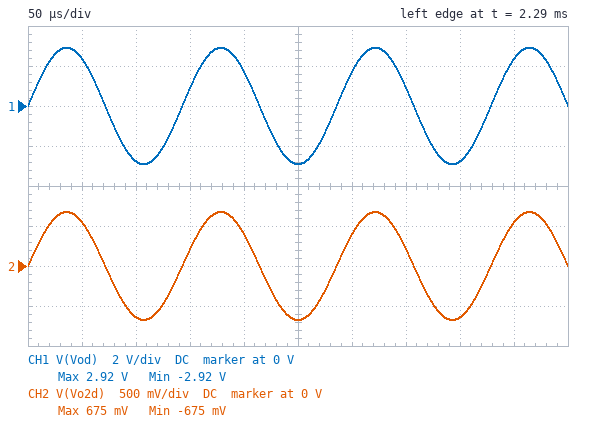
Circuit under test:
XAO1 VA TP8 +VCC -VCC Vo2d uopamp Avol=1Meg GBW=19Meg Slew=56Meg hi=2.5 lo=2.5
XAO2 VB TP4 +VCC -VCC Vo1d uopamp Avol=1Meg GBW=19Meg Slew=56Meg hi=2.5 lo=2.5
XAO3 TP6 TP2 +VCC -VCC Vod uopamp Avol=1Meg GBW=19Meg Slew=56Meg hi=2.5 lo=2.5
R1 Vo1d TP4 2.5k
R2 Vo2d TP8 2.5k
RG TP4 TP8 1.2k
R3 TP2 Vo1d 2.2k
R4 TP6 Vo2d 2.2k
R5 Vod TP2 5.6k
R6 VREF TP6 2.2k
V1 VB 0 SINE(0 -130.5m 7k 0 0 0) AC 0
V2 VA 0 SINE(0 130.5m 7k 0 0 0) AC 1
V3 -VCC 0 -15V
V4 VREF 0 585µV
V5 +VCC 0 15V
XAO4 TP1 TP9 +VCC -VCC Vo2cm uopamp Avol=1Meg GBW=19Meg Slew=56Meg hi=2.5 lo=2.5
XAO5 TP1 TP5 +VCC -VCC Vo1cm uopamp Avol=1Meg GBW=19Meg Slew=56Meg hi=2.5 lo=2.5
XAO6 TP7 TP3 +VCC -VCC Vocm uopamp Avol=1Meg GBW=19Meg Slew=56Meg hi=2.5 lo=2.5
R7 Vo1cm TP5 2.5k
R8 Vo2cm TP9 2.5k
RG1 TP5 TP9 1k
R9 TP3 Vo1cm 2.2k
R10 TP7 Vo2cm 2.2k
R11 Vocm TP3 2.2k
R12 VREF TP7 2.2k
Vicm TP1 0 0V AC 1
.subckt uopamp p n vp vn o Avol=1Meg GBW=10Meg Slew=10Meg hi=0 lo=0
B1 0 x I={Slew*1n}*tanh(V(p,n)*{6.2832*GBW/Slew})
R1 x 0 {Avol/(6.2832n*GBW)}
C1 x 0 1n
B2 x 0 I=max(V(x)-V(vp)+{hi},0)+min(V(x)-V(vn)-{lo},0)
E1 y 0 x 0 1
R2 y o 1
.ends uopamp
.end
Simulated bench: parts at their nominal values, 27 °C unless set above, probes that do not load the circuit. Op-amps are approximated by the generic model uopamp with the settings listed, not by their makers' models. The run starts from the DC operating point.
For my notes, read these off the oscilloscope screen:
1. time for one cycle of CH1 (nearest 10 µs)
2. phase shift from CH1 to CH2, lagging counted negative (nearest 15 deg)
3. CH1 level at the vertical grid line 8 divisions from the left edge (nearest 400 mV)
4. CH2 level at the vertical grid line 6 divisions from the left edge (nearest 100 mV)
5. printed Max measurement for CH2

140 µs
0 deg
-2.8 V
400 mV
675 mV
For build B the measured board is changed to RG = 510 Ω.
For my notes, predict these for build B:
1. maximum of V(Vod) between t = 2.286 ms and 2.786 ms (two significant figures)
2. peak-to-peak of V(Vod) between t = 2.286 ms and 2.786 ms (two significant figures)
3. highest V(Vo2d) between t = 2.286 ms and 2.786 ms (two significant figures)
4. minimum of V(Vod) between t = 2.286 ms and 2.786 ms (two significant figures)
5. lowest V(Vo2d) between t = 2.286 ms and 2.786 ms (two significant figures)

6.1 V
12 V
1.4 V
-6.1 V
-1.4 V
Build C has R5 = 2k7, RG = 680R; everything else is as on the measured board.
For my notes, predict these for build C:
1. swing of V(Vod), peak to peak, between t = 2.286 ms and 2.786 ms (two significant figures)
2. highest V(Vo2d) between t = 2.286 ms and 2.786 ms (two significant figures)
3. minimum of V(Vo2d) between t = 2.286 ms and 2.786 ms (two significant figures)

5.1 V
1.1 V
-1.1 V
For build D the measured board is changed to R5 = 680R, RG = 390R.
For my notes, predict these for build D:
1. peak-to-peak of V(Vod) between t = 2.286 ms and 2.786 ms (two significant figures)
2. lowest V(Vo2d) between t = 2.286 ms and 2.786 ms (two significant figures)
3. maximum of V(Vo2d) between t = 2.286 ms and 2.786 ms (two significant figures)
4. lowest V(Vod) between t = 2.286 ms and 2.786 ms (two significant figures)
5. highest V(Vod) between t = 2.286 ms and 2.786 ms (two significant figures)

3.5 V
-1.8 V
1.8 V
-1.7 V
1.7 V
